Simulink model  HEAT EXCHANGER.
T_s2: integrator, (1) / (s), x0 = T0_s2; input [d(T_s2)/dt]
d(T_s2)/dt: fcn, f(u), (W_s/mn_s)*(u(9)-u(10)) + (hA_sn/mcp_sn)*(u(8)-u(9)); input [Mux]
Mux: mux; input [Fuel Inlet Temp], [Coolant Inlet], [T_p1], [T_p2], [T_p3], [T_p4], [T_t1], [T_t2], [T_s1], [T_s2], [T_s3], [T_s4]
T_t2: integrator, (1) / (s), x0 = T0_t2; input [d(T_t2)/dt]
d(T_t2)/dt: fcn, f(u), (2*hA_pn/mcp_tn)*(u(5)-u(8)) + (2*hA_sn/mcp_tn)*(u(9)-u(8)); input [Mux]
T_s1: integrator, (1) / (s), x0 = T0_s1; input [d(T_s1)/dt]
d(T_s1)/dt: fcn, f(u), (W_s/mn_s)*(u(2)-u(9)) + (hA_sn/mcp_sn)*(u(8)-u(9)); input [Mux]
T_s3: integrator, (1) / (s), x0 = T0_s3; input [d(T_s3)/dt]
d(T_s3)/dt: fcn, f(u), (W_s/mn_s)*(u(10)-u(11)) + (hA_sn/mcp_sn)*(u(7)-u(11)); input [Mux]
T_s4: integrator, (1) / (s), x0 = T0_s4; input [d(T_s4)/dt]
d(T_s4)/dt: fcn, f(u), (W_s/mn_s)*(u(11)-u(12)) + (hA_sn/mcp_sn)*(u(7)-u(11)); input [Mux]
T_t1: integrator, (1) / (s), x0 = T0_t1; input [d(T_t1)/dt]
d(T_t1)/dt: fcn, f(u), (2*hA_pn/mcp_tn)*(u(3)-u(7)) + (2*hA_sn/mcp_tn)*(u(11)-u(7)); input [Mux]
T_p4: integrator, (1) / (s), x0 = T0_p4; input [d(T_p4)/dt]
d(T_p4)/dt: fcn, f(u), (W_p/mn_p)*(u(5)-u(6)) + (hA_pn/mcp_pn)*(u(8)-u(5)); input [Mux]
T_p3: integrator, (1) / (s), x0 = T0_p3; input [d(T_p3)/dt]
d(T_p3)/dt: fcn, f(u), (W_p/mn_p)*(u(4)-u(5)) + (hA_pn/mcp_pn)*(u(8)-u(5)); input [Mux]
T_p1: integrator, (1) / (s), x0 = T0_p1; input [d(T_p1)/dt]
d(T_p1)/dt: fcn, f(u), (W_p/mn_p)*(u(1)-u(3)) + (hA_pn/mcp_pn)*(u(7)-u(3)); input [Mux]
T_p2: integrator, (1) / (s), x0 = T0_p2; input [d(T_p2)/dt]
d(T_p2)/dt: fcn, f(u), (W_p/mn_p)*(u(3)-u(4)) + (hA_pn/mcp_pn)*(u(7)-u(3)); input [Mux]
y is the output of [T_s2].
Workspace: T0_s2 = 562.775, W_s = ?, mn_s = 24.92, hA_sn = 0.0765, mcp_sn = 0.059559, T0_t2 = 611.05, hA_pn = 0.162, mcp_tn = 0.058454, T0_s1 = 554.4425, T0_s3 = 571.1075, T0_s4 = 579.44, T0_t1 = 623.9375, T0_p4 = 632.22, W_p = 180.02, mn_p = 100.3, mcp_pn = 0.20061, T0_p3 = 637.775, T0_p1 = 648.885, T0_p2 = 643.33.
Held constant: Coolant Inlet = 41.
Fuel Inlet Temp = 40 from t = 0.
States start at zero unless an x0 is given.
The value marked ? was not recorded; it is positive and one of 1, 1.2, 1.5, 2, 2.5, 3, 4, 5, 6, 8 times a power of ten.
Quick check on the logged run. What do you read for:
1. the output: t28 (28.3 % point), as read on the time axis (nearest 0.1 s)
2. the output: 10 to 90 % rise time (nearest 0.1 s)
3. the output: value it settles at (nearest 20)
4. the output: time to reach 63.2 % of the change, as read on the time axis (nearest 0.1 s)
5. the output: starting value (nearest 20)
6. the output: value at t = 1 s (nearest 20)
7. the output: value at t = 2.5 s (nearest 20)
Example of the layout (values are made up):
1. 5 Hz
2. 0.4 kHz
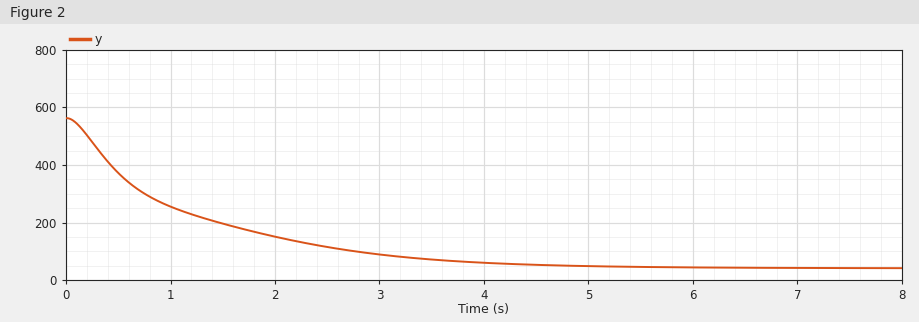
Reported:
1. 0.4 s
2. 2.7 s
3. 40
4. 1.2 s
5. 560
6. 260
7. 120
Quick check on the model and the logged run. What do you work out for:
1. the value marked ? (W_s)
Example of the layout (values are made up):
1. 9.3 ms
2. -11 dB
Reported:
1. 100
